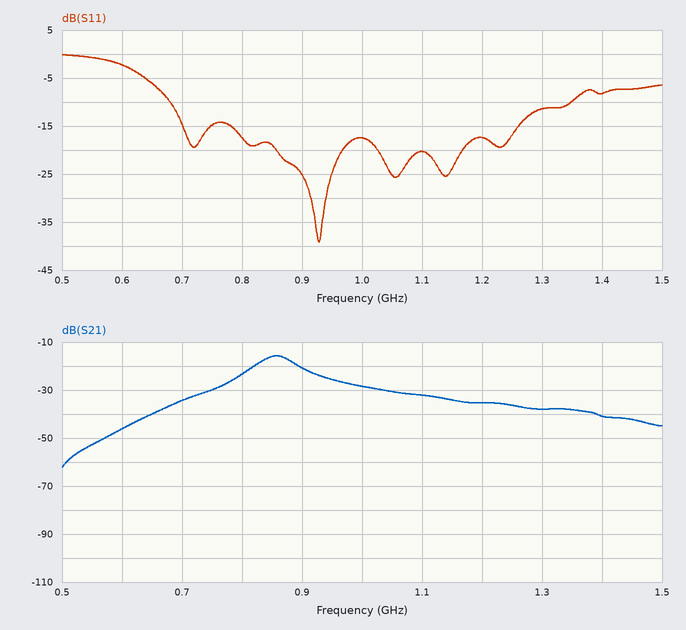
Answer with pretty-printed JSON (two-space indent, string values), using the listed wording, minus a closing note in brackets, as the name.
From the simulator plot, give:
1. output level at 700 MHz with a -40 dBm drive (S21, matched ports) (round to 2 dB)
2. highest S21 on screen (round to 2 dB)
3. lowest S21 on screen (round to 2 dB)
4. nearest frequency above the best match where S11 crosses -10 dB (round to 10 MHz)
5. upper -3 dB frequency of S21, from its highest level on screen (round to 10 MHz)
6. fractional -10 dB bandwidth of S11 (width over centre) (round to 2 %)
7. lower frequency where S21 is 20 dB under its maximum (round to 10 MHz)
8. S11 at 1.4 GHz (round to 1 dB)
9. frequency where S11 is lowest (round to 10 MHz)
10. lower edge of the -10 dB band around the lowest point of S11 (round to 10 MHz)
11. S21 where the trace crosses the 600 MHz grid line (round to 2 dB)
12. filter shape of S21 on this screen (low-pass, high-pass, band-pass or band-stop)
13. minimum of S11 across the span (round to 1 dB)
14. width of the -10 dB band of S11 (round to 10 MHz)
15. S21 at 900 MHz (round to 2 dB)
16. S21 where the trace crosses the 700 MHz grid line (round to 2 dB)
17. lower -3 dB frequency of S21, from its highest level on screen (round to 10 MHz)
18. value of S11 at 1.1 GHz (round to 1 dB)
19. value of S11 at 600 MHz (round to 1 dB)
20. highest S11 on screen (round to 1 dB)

{
  "output level at 700 MHz with a -40 dBm drive (S21, matched ports)": "-74 dBm",
  "highest S21 on screen": "-16 dB",
  "lowest S21 on screen": "-62 dB",
  "nearest frequency above the best match where S11 crosses -10 dB": "1.35 GHz",
  "upper -3 dB frequency of S21, from its highest level on screen": "890 MHz",
  "fractional -10 dB bandwidth of S11 (width over centre)": "66 %",
  "lower frequency where S21 is 20 dB under its maximum": "690 MHz",
  "S11 at 1.4 GHz": "-8 dB",
  "frequency where S11 is lowest": "930 MHz",
  "lower edge of the -10 dB band around the lowest point of S11": "680 MHz",
  "S21 where the trace crosses the 600 MHz grid line": "-46 dB",
  "filter shape of S21 on this screen": "band-pass",
  "minimum of S11 across the span": "-39 dB",
  "width of the -10 dB band of S11": "670 MHz",
  "S21 at 900 MHz": "-20 dB",
  "S21 where the trace crosses the 700 MHz grid line": "-34 dB",
  "lower -3 dB frequency of S21, from its highest level on screen": "830 MHz",
  "value of S11 at 1.1 GHz": "-20 dB",
  "value of S11 at 600 MHz": "-2 dB",
  "highest S11 on screen": "0 dB"
}
